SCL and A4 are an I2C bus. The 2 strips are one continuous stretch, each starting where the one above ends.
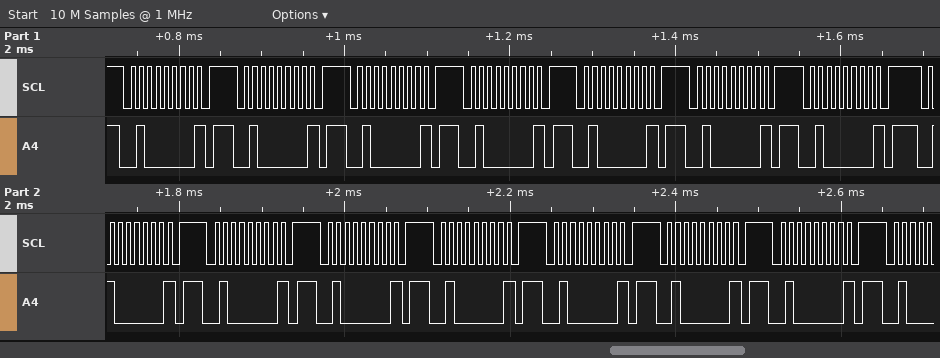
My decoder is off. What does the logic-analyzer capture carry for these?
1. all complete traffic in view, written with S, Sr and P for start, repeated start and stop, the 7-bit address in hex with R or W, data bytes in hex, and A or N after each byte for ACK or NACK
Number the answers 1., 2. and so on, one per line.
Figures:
1. S 20W N P S 20W N P S 20W N P S 20W N P S 20W N P S 20W N P S 20W N P S 20W N P S 20W N P S 20W N P S 20W N P S 20W N P S 20W N P S 20W N P
